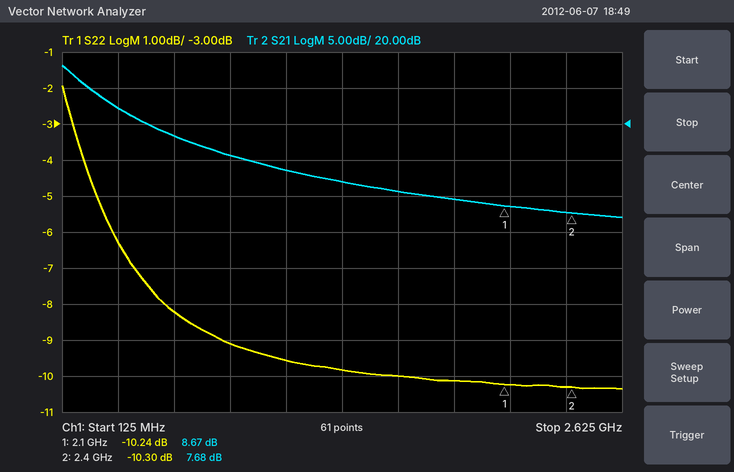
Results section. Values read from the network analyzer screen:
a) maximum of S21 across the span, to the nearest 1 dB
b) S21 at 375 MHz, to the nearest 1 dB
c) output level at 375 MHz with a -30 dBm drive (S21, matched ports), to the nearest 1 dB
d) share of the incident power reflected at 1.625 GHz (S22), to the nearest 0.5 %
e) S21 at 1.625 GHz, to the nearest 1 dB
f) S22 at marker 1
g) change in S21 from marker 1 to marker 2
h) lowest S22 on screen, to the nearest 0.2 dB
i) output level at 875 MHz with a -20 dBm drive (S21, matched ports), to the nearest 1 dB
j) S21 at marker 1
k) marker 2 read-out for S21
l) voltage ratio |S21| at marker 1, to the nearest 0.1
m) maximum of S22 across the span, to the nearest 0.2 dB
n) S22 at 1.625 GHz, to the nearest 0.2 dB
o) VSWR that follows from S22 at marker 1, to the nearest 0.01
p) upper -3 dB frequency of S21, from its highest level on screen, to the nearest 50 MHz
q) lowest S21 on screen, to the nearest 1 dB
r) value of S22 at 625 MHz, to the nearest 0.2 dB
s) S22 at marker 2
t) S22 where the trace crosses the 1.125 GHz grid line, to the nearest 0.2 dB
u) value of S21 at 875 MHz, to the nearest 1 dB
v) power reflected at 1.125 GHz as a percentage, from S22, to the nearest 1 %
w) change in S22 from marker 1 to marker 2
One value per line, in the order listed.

28 dB
22 dB
-8 dBm
10.0 %
11 dB
-10.24 dB
-0.99 dB
-10.4 dB
-4 dBm
8.67 dB
7.68 dB
2.7
-2.0 dB
-10.0 dB
1.89
250 MHz
7 dB
-8.2 dB
-10.30 dB
-9.6 dB
16 dB
11 %
-0.06 dB
